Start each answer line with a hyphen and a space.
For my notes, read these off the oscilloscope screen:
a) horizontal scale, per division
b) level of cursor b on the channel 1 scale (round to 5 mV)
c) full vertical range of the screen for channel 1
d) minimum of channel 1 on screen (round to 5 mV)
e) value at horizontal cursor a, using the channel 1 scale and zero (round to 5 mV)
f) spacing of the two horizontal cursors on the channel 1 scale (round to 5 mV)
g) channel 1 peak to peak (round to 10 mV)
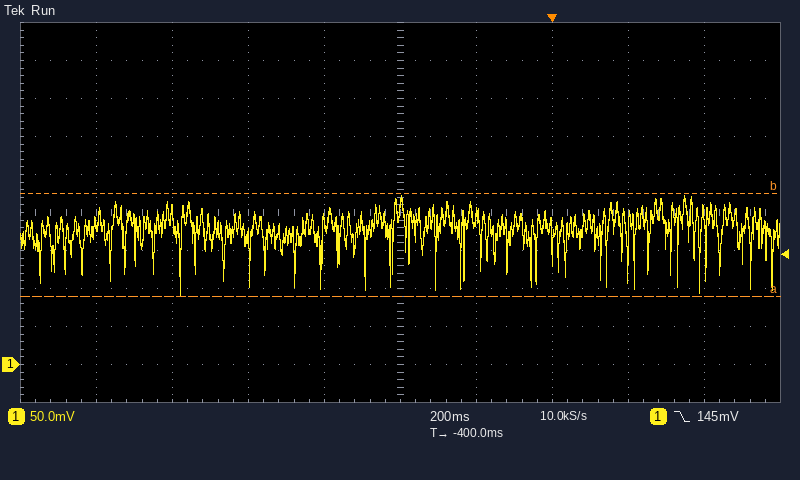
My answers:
- 200 ms
- 225 mV
- 500 mV
- 90 mV
- 90 mV
- 135 mV
- 130 mV
